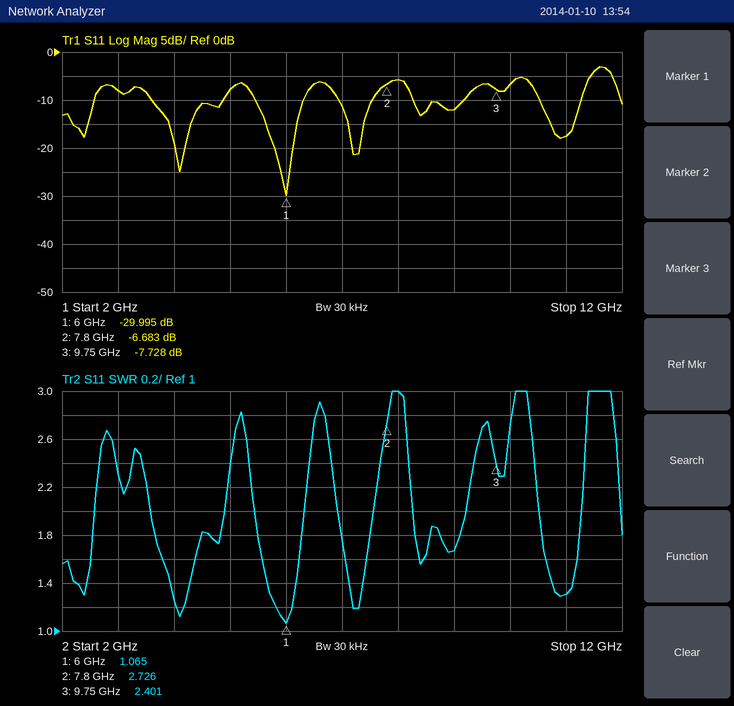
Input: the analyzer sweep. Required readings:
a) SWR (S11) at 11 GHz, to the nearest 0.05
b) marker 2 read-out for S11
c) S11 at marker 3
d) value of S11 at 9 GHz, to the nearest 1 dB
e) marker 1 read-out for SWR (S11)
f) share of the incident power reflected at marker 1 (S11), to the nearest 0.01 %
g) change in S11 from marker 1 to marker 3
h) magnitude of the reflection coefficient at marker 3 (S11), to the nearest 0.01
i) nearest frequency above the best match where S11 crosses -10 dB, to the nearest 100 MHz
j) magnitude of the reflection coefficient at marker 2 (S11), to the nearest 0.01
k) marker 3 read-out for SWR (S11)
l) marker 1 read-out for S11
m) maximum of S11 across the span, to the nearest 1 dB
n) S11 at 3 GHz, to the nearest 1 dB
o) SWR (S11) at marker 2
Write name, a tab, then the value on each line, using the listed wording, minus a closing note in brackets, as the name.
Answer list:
SWR (S11) at 11 GHz, to the nearest 0.05	1.30
marker 2 read-out for S11	-6.683 dB
S11 at marker 3	-7.728 dB
value of S11 at 9 GHz, to the nearest 1 dB	-12 dB
marker 1 read-out for SWR	1.065
share of the incident power reflected at marker 1 (S11), to the nearest 0.01 %	0.10 %
change in S11 from marker 1 to marker 3	22.267 dB
magnitude of the reflection coefficient at marker 3 (S11), to the nearest 0.01	0.41
nearest frequency above the best match where S11 crosses -10 dB, to the nearest 100 MHz	6.3 GHz
magnitude of the reflection coefficient at marker 2 (S11), to the nearest 0.01	0.46
marker 3 read-out for SWR	2.401
marker 1 read-out for S11	-29.995 dB
maximum of S11 across the span, to the nearest 1 dB	-3 dB
S11 at 3 GHz, to the nearest 1 dB	-8 dB
SWR (S11) at marker 2	2.726
